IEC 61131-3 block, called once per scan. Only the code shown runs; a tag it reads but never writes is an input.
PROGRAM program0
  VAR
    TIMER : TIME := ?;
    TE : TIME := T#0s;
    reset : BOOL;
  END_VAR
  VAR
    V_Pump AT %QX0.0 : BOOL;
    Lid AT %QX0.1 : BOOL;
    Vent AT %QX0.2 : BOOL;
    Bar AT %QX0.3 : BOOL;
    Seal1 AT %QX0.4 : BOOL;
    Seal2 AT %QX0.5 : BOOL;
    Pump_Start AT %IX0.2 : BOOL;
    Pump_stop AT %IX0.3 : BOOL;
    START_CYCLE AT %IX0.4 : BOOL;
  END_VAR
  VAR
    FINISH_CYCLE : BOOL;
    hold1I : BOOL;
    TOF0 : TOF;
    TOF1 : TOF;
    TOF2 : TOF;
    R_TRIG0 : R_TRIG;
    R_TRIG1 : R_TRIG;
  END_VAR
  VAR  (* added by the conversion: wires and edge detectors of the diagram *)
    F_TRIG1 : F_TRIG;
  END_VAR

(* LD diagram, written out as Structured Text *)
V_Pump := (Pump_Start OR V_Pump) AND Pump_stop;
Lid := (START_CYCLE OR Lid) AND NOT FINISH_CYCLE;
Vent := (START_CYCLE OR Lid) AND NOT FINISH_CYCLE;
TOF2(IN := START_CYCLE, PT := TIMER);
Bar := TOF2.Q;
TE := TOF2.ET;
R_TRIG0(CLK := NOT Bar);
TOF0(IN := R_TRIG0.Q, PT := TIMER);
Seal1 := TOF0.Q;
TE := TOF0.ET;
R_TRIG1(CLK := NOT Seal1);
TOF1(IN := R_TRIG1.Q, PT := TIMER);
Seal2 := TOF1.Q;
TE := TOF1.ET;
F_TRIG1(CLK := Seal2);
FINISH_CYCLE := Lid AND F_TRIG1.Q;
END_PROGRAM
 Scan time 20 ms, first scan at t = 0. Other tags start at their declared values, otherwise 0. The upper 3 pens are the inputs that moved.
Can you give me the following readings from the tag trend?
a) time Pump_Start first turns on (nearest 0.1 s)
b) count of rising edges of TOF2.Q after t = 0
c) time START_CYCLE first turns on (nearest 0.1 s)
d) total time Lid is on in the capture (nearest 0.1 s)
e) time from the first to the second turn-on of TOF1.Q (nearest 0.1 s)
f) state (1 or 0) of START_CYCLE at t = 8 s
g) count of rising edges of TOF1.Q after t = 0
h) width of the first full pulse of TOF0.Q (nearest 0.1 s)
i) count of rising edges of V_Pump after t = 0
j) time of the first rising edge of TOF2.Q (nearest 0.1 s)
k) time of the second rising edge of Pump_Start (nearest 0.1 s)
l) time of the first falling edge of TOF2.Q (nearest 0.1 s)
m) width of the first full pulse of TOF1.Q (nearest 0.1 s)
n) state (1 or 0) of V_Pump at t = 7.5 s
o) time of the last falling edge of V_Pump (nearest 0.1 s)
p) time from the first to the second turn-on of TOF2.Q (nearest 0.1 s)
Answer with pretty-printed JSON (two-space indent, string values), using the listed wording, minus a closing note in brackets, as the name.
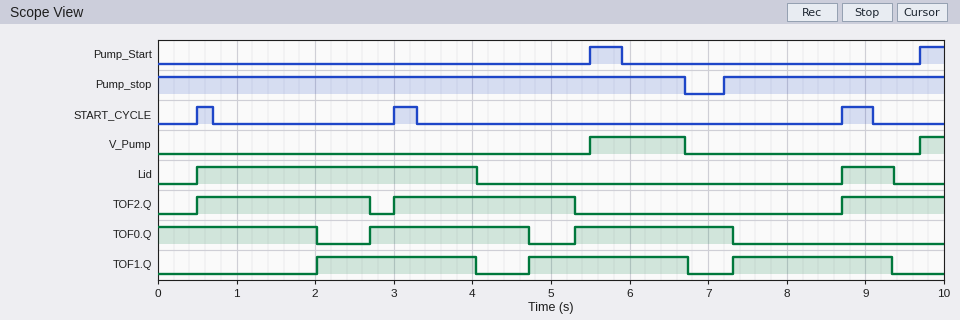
{
  "time Pump_Start first turns on": "5.5 s",
  "count of rising edges of TOF2.Q after t = 0": "3",
  "time START_CYCLE first turns on": "0.5 s",
  "total time Lid is on in the capture": "4.2 s",
  "time from the first to the second turn-on of TOF1.Q": "2.7 s",
  "state (1 or 0) of START_CYCLE at t = 8 s": "0",
  "count of rising edges of TOF1.Q after t = 0": "3",
  "width of the first full pulse of TOF0.Q": "2.0 s",
  "count of rising edges of V_Pump after t = 0": "2",
  "time of the first rising edge of TOF2.Q": "0.5 s",
  "time of the second rising edge of Pump_Start": "9.7 s",
  "time of the first falling edge of TOF2.Q": "2.7 s",
  "width of the first full pulse of TOF1.Q": "2.0 s",
  "state (1 or 0) of V_Pump at t = 7.5 s": "0",
  "time of the last falling edge of V_Pump": "6.7 s",
  "time from the first to the second turn-on of TOF2.Q": "2.5 s"
}
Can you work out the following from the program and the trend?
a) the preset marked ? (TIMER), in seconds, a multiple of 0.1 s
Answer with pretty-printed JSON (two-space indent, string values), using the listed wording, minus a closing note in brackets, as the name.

{
  "the preset marked ? (TIMER), in seconds, a multiple of 0.1 s": "2.0 s"
}
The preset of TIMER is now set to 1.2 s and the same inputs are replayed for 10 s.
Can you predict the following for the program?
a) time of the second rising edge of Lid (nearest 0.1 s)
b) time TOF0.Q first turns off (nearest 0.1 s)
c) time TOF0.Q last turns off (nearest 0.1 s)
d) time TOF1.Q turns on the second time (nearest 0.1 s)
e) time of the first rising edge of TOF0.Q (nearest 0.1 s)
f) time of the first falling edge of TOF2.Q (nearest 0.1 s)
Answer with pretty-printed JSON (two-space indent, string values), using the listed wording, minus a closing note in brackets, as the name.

{
  "time of the second rising edge of Lid": "3.0 s",
  "time TOF0.Q first turns off": "1.2 s",
  "time TOF0.Q last turns off": "5.7 s",
  "time TOF1.Q turns on the second time": "3.1 s",
  "time of the first rising edge of TOF0.Q": "1.9 s",
  "time of the first falling edge of TOF2.Q": "1.9 s"
}
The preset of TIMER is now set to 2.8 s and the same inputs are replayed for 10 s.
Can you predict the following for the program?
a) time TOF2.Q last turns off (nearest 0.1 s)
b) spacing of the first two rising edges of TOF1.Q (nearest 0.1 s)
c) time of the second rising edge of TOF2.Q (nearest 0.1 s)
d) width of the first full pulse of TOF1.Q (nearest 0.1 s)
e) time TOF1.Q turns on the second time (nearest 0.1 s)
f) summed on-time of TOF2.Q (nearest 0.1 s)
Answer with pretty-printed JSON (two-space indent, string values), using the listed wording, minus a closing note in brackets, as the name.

{
  "time TOF2.Q last turns off": "6.1 s",
  "spacing of the first two rising edges of TOF1.Q": "6.1 s",
  "time of the second rising edge of TOF2.Q": "8.7 s",
  "width of the first full pulse of TOF1.Q": "2.8 s",
  "time TOF1.Q turns on the second time": "8.9 s",
  "summed on-time of TOF2.Q": "6.9 s"
}
